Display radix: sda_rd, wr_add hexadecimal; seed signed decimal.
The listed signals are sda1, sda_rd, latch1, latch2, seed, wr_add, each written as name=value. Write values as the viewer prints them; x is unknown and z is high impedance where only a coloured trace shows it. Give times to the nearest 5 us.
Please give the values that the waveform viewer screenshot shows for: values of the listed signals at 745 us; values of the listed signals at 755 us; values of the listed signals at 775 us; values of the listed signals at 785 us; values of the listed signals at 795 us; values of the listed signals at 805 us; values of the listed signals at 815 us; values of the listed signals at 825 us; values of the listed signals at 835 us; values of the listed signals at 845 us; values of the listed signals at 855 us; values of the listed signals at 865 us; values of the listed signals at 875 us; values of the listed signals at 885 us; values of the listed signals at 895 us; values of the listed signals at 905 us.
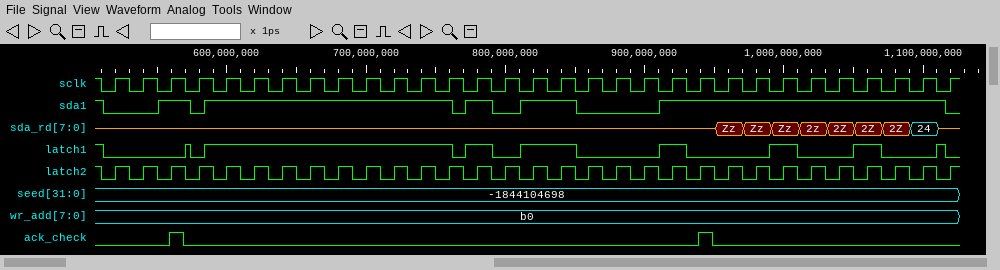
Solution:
sda1=1, sda_rd=z, latch1=1, latch2=1, seed=-1844104698, wr_add=b0
sda1=1, sda_rd=z, latch1=1, latch2=0, seed=-1844104698, wr_add=b0
sda1=1, sda_rd=z, latch1=1, latch2=0, seed=-1844104698, wr_add=b0
sda1=1, sda_rd=z, latch1=1, latch2=1, seed=-1844104698, wr_add=b0
sda1=0, sda_rd=z, latch1=0, latch2=0, seed=-1844104698, wr_add=b0
sda1=0, sda_rd=z, latch1=0, latch2=1, seed=-1844104698, wr_add=b0
sda1=1, sda_rd=z, latch1=1, latch2=0, seed=-1844104698, wr_add=b0
sda1=1, sda_rd=z, latch1=1, latch2=1, seed=-1844104698, wr_add=b0
sda1=1, sda_rd=z, latch1=1, latch2=0, seed=-1844104698, wr_add=b0
sda1=1, sda_rd=z, latch1=1, latch2=1, seed=-1844104698, wr_add=b0
sda1=0, sda_rd=z, latch1=0, latch2=0, seed=-1844104698, wr_add=b0
sda1=0, sda_rd=z, latch1=0, latch2=1, seed=-1844104698, wr_add=b0
sda1=0, sda_rd=z, latch1=0, latch2=0, seed=-1844104698, wr_add=b0
sda1=0, sda_rd=z, latch1=0, latch2=1, seed=-1844104698, wr_add=b0
sda1=0, sda_rd=z, latch1=0, latch2=0, seed=-1844104698, wr_add=b0
sda1=0, sda_rd=z, latch1=0, latch2=1, seed=-1844104698, wr_add=b0
